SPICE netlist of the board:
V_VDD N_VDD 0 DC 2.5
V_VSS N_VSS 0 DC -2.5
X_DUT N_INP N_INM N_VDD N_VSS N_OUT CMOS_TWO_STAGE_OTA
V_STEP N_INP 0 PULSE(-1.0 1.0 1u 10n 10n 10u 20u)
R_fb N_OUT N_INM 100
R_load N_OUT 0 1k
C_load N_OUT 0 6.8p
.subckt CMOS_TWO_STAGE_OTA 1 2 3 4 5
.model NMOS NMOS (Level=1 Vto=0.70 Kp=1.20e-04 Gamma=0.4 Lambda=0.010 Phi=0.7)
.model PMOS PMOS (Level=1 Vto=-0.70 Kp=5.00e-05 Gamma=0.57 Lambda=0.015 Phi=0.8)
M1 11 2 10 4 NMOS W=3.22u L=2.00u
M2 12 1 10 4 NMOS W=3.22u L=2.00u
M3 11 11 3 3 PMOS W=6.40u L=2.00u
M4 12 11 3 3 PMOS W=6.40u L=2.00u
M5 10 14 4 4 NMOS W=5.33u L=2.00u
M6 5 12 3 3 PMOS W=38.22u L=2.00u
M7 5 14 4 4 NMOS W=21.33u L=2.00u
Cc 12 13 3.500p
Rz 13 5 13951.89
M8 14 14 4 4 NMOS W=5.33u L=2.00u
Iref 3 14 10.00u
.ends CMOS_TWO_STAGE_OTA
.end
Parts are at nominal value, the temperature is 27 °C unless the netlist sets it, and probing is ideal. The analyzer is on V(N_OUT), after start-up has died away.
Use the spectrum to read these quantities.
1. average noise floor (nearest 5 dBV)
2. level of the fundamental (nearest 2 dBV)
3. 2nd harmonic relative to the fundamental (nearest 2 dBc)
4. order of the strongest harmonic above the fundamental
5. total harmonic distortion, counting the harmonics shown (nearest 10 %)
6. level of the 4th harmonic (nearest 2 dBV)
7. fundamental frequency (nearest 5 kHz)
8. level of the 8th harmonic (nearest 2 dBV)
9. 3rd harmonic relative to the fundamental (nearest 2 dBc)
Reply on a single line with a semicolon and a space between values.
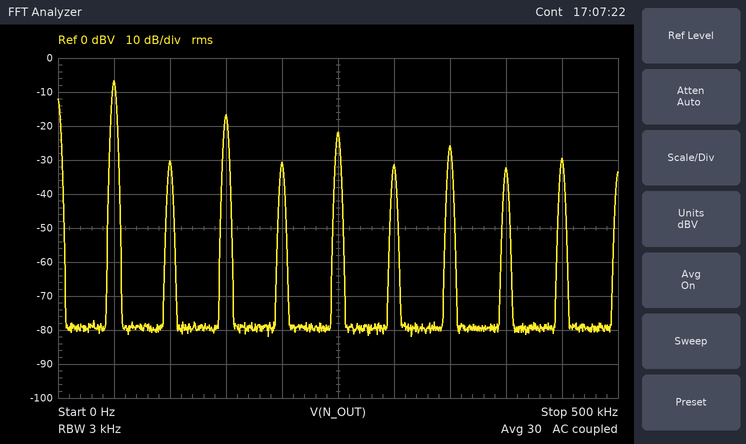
-80 dBV; -6 dBV; -24 dBc; 3; 40 %; -30 dBV; 50 kHz; -32 dBV; -10 dBc
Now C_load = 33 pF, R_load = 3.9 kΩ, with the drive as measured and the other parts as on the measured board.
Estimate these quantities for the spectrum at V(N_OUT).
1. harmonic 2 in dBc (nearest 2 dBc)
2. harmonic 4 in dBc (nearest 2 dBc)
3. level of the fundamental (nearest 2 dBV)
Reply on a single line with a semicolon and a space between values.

-26 dBc; -26 dBc; -6 dBV
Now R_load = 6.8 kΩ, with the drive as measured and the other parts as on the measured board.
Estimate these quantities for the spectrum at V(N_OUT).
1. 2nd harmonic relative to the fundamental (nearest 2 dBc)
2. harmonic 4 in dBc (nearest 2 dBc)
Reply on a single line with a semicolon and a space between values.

-26 dBc; -26 dBc
